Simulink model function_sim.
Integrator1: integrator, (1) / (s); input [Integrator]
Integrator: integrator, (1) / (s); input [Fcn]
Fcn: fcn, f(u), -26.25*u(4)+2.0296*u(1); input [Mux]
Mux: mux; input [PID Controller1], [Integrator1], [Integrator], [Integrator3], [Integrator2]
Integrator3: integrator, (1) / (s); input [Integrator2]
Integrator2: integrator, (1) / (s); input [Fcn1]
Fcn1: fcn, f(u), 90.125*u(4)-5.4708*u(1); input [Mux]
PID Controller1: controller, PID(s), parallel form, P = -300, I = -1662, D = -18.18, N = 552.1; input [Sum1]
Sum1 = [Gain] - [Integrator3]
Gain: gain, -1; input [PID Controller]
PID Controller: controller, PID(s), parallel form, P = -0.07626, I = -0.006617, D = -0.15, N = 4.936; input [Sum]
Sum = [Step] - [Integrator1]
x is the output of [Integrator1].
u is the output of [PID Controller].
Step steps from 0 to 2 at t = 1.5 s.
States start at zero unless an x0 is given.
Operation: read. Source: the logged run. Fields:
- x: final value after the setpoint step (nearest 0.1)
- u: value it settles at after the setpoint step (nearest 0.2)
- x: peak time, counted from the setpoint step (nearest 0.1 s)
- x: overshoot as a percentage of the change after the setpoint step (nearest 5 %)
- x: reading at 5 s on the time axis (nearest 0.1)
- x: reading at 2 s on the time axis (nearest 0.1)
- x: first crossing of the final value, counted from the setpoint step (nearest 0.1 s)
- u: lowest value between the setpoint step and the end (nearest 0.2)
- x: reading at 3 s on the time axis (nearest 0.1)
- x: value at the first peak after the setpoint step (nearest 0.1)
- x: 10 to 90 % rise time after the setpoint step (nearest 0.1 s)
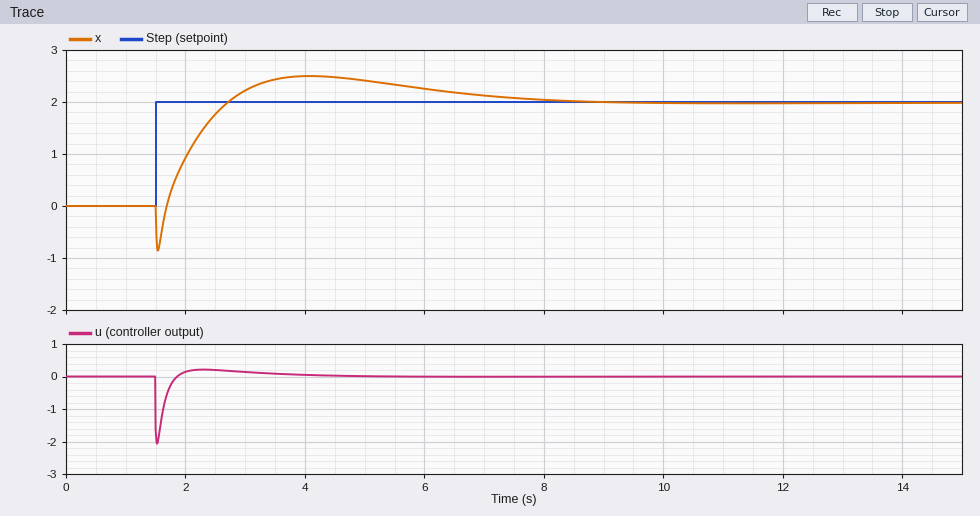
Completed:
2.0
0.0
2.6 s
25 %
2.4
0.9
1.2 s
-2.0
2.2
2.5
0.8 s
